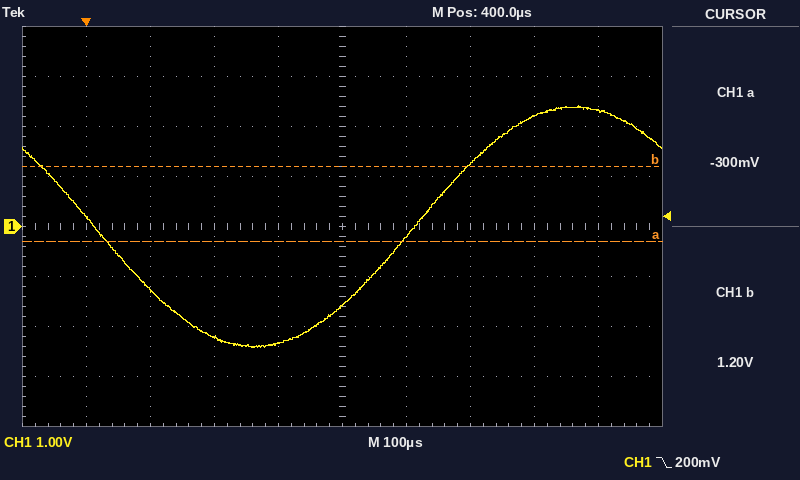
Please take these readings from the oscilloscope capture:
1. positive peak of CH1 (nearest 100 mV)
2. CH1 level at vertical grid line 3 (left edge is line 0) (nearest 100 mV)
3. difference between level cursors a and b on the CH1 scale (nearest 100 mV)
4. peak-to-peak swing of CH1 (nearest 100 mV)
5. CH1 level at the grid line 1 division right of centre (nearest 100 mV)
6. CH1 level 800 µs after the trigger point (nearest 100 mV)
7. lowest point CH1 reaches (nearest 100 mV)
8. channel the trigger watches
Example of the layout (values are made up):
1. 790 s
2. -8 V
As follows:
1. 2.4 V
2. -2.2 V
3. 1.5 V
4. 4.8 V
5. -200 mV
6. 2.3 V
7. -2.4 V
8. CH1
